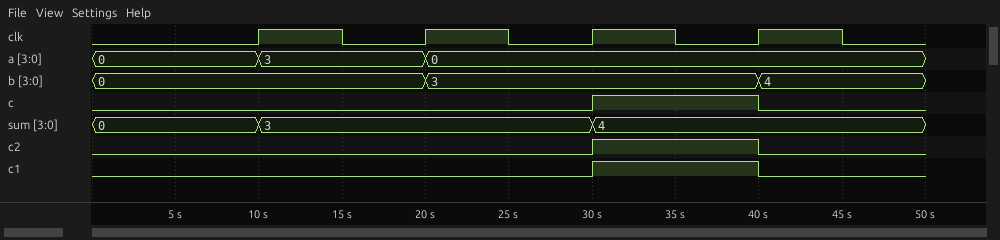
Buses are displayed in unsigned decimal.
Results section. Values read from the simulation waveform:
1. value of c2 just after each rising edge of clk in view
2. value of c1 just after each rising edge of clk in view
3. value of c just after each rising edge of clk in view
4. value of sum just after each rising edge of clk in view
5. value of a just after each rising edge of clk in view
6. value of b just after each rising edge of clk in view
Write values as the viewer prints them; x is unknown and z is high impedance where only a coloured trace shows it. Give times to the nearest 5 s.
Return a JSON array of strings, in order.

["0 0 1 0", "0 0 1 0", "0 0 1 0", "3, 3, 4, 4", "3, 0, 0, 0", "0, 3, 3, 4"]
